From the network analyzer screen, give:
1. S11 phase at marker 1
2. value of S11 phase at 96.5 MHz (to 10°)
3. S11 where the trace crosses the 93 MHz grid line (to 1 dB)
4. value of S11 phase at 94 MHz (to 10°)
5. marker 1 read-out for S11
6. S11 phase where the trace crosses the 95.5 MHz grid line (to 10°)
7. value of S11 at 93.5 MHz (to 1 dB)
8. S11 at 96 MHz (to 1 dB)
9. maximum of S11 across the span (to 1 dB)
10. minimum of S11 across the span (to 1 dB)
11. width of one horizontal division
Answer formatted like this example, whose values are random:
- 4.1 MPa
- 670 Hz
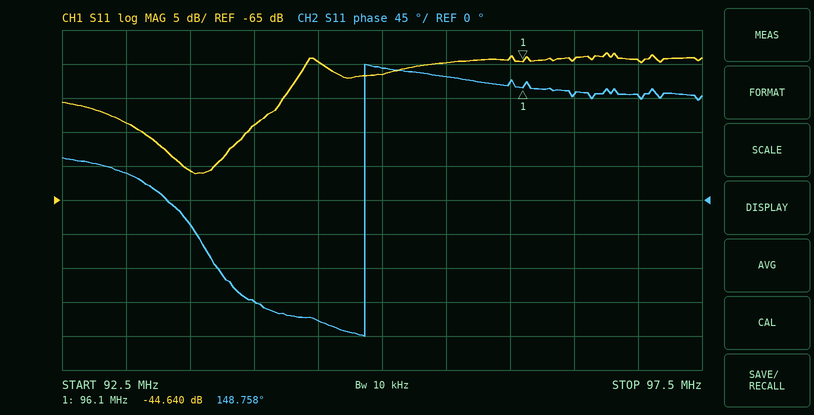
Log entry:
- 148.758°
- 140°
- -54 dB
- -130°
- -44.640 dB
- 160°
- -61 dB
- -44 dB
- -43 dB
- -61 dB
- 500 kHz
